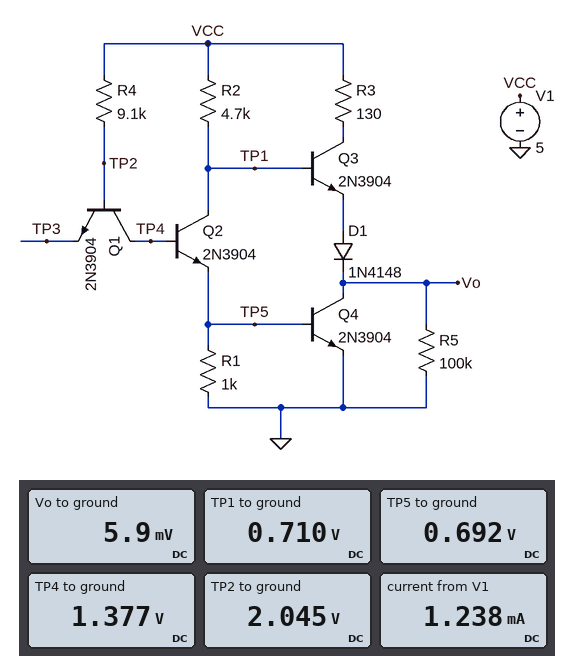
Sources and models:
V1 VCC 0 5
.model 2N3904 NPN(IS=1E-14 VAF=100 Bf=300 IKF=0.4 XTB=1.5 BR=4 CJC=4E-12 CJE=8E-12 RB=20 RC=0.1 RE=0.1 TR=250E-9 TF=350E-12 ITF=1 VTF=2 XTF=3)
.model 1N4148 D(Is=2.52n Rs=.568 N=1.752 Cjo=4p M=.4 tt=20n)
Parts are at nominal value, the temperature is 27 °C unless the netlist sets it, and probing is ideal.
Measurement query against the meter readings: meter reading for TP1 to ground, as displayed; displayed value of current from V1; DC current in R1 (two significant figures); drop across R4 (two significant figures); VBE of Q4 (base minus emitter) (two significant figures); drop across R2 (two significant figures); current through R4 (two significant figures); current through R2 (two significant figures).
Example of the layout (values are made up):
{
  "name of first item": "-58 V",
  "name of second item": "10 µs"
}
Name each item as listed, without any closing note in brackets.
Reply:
{
  "meter reading for TP1 to ground, as displayed": "0.710 V",
  "displayed value of current from V1": "1.238 mA",
  "DC current in R1": "690 µA",
  "drop across R4": "3.0 V",
  "VBE of Q4 (base minus emitter)": "690 mV",
  "drop across R2": "4.3 V",
  "current through R4": "320 µA",
  "current through R2": "910 µA"
}
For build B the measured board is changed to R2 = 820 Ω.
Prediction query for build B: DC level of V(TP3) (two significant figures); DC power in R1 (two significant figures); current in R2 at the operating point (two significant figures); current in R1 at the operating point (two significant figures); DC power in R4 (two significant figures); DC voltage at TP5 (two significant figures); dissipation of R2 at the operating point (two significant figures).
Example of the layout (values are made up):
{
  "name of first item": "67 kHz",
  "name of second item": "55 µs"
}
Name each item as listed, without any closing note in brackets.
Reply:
{
  "DC level of V(TP3)": "1.5 V",
  "DC power in R1": "680 µW",
  "current in R2 at the operating point": "5.0 mA",
  "current in R1 at the operating point": "830 µA",
  "DC power in R4": "860 µW",
  "DC voltage at TP5": "830 mV",
  "dissipation of R2 at the operating point": "21 mW"
}
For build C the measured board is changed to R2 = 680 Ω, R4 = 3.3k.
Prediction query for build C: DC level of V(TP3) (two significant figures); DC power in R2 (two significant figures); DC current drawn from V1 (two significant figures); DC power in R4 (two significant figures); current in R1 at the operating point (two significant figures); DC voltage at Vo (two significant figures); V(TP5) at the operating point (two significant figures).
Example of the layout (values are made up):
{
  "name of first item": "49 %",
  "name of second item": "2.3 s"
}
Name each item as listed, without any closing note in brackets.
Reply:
{
  "DC level of V(TP3)": "1.6 V",
  "DC power in R2": "25 mW",
  "DC current drawn from V1": "6.9 mA",
  "DC power in R4": "2.2 mW",
  "current in R1 at the operating point": "860 µA",
  "DC voltage at Vo": "6.8 mV",
  "V(TP5) at the operating point": "860 mV"
}
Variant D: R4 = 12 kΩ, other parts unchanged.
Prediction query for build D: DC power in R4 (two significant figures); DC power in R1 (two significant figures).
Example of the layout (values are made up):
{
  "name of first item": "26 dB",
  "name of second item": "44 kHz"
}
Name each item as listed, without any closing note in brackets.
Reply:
{
  "DC power in R4": "740 µW",
  "DC power in R1": "470 µW"
}
